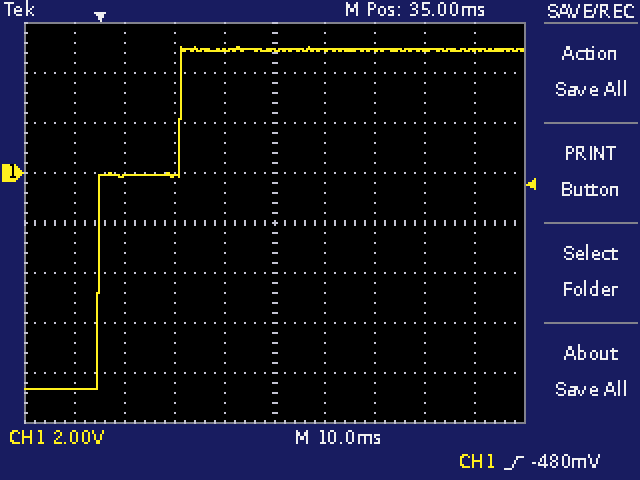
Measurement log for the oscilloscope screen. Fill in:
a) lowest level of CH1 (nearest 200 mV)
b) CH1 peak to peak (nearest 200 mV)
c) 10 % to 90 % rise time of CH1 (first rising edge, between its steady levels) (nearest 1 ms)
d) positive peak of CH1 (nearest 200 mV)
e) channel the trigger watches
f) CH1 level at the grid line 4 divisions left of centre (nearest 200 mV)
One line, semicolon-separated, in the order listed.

-8.6 V; 13.6 V; 17 ms; 5.0 V; CH1; -8.6 V
